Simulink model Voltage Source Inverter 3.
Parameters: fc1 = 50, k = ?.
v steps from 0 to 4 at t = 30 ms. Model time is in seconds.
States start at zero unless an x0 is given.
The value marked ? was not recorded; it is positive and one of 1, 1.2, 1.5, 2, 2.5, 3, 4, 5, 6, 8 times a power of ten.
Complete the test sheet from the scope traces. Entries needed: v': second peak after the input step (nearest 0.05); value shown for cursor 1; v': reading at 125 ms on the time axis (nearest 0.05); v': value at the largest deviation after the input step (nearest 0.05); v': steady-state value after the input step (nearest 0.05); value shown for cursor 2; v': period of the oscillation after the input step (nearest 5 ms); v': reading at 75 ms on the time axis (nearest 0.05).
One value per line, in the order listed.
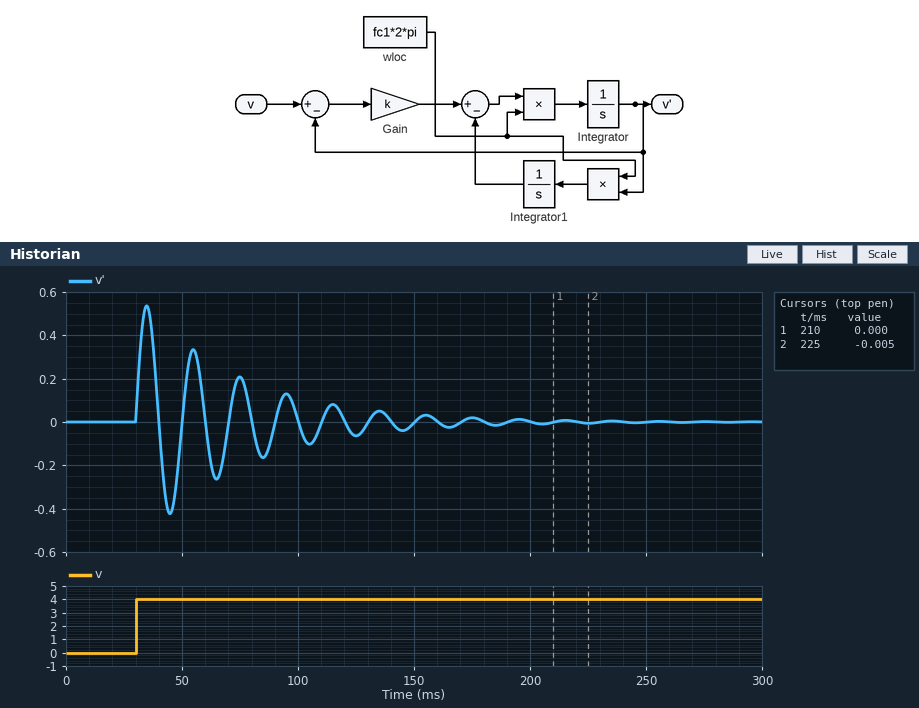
0.35
0.000
-0.05
0.55
0.00
-0.005
20 ms
0.20
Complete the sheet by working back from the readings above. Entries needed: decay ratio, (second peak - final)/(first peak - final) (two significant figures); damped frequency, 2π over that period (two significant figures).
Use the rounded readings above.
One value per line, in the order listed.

0.64
0.31 rad/ms
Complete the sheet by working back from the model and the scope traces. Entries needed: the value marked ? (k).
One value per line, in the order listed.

0.15
